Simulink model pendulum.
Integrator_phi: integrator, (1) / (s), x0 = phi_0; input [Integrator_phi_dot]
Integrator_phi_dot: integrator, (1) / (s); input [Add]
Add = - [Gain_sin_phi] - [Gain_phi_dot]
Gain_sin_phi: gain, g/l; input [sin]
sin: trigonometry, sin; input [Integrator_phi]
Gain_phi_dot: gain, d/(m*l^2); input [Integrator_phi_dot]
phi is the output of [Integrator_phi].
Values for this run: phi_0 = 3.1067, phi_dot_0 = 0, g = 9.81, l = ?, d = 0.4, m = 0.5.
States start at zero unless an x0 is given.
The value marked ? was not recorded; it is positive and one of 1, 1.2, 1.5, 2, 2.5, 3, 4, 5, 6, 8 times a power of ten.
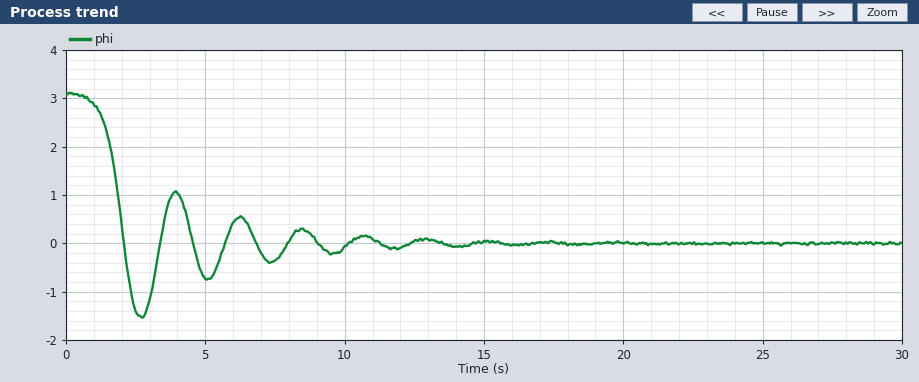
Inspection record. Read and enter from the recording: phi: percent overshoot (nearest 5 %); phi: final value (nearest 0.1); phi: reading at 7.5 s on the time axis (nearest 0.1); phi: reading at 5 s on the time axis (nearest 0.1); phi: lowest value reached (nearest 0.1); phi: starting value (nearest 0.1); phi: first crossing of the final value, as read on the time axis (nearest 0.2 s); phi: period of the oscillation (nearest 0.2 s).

50 %
0.0
-0.4
-0.7
-1.5
3.1
2.0 s
2.4 s
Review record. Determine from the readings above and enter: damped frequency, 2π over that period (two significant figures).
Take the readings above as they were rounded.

2.6 rad/s
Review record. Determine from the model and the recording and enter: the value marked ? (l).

1.2
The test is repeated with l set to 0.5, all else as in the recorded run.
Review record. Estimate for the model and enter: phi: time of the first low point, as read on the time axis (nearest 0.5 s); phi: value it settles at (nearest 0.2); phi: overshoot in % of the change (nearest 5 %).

2.0 s
0.0
15 %
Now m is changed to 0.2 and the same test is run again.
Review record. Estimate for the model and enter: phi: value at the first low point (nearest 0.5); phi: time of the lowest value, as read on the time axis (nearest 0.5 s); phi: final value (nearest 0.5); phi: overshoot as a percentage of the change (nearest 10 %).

-1.0
3.0 s
0.0
30 %
